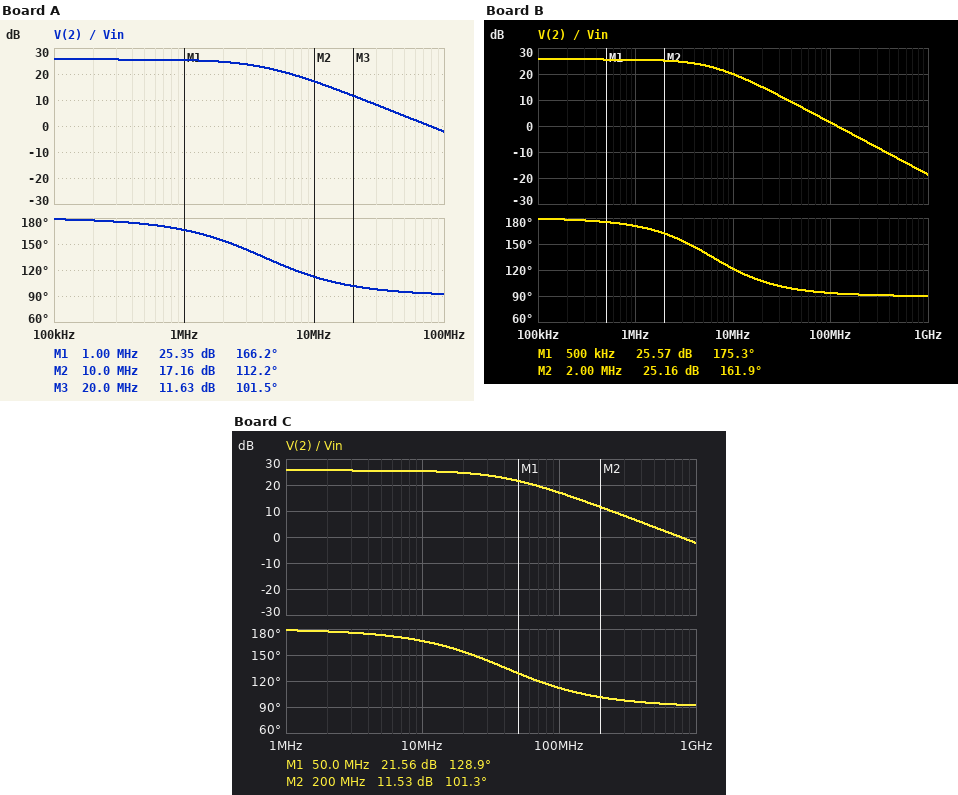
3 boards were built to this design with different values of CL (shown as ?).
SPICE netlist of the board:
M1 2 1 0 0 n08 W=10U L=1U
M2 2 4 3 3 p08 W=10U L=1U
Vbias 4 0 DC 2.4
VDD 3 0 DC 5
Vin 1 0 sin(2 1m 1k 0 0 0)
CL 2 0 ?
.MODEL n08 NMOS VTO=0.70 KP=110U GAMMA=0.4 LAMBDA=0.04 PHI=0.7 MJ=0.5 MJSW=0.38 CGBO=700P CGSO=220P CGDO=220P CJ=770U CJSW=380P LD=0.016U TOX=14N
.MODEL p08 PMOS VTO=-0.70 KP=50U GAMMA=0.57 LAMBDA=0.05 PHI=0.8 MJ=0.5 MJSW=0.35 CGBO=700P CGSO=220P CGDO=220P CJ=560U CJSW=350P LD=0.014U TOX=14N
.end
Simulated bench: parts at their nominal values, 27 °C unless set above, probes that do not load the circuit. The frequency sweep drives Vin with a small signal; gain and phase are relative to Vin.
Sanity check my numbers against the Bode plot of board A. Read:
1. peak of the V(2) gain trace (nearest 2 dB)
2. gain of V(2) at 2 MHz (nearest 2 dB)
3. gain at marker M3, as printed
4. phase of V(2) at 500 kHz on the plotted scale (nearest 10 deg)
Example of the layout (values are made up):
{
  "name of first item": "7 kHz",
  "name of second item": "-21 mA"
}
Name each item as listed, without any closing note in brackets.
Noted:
{
  "peak of the V(2) gain trace": "26 dB",
  "gain of V(2) at 2 MHz": "24 dB",
  "gain at marker M3, as printed": "11.63 dB",
  "phase of V(2) at 500 kHz on the plotted scale": "170 deg"
}
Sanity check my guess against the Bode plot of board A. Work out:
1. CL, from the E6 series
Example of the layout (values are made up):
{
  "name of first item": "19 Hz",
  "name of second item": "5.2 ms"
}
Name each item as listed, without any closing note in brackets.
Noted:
{
  "CL, from the E6 series": "3.3 pF"
}
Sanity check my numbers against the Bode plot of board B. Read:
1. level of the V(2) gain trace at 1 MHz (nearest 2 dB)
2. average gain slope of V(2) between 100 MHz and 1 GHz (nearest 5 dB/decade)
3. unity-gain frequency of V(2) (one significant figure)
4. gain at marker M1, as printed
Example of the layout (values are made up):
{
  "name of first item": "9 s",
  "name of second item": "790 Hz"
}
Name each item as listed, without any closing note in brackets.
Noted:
{
  "level of the V(2) gain trace at 1 MHz": "26 dB",
  "average gain slope of V(2) between 100 MHz and 1 GHz": "-20 dB/decade",
  "unity-gain frequency of V(2)": "100 MHz",
  "gain at marker M1, as printed": "25.57 dB"
}
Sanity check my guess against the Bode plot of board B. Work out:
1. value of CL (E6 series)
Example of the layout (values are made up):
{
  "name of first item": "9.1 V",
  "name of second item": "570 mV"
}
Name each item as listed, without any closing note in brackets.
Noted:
{
  "value of CL": "2.2 pF"
}
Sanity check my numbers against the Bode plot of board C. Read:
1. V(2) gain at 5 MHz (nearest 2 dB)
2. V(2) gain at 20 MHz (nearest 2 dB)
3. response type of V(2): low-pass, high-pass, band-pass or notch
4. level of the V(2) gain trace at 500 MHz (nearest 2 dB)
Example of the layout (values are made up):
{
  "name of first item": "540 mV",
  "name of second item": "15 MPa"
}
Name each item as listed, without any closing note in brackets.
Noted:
{
  "V(2) gain at 5 MHz": "26 dB",
  "V(2) gain at 20 MHz": "24 dB",
  "response type of V(2): low-pass, high-pass, band-pass or notch": "low-pass",
  "level of the V(2) gain trace at 500 MHz": "4 dB"
}
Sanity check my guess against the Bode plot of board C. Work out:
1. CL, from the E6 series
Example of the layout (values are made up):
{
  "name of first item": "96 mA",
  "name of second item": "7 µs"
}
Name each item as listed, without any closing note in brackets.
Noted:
{
  "CL, from the E6 series": "330 fF"
}
